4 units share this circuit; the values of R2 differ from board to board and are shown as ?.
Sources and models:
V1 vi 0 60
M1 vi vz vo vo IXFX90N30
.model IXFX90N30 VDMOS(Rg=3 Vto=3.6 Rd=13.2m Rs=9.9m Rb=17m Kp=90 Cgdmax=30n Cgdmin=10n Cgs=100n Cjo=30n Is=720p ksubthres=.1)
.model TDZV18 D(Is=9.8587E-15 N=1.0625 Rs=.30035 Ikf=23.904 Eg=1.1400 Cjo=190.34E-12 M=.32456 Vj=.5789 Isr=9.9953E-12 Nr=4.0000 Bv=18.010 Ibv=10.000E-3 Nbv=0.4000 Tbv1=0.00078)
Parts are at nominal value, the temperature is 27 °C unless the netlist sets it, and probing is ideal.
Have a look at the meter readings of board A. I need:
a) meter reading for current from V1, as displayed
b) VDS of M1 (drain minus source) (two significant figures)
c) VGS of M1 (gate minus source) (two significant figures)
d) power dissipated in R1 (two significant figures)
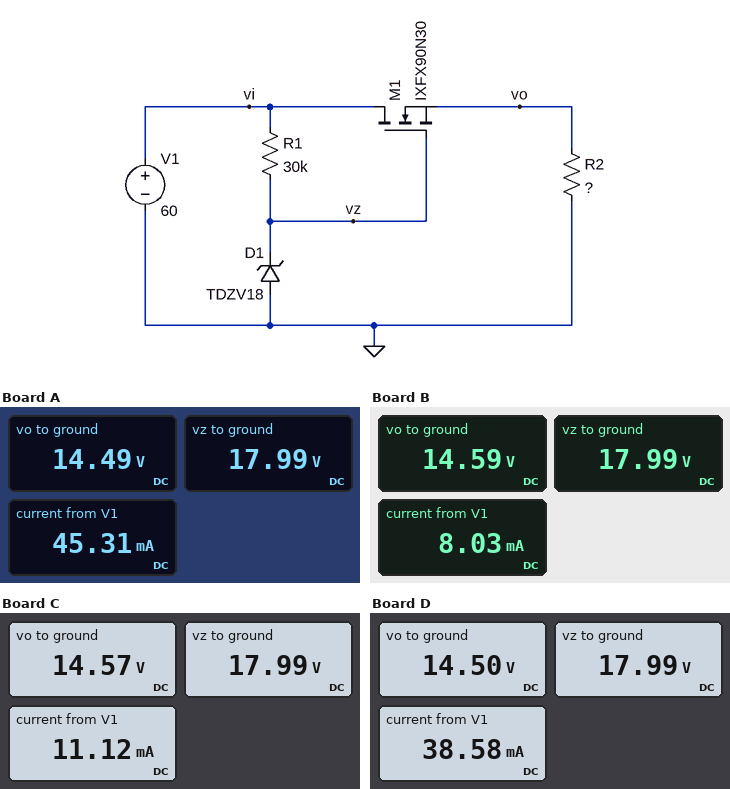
45.31 mA
46 V
3.5 V
59 mW
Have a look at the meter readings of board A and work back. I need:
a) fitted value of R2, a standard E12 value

330 Ω
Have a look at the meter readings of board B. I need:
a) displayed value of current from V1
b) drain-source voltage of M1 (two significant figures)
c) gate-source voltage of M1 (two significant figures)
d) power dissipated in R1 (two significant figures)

8.03 mA
45 V
3.4 V
59 mW
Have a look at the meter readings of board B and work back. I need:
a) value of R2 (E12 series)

2.2 kΩ
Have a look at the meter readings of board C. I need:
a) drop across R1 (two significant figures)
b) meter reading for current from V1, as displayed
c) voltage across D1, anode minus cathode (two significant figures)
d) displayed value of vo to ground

42 V
11.12 mA
-18 V
14.57 V
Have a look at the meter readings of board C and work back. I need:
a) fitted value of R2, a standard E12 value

1.5 kΩ
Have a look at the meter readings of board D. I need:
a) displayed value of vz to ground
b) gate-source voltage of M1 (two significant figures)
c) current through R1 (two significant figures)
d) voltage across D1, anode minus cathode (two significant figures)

17.99 V
3.5 V
1.4 mA
-18 V
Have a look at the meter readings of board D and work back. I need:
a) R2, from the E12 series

390 Ω
